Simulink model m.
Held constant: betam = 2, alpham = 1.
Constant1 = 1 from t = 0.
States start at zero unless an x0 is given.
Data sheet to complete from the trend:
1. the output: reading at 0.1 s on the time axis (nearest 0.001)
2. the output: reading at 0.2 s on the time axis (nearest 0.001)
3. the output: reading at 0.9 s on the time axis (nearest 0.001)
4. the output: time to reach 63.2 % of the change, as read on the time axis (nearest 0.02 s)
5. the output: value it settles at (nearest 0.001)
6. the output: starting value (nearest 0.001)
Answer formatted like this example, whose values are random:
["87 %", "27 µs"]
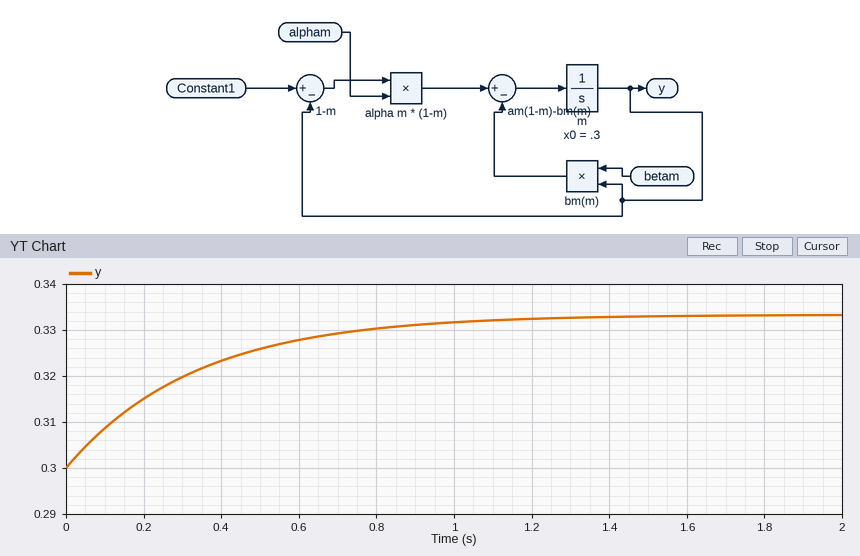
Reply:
["0.309", "0.315", "0.331", "0.34 s", "0.333", "0.300"]
